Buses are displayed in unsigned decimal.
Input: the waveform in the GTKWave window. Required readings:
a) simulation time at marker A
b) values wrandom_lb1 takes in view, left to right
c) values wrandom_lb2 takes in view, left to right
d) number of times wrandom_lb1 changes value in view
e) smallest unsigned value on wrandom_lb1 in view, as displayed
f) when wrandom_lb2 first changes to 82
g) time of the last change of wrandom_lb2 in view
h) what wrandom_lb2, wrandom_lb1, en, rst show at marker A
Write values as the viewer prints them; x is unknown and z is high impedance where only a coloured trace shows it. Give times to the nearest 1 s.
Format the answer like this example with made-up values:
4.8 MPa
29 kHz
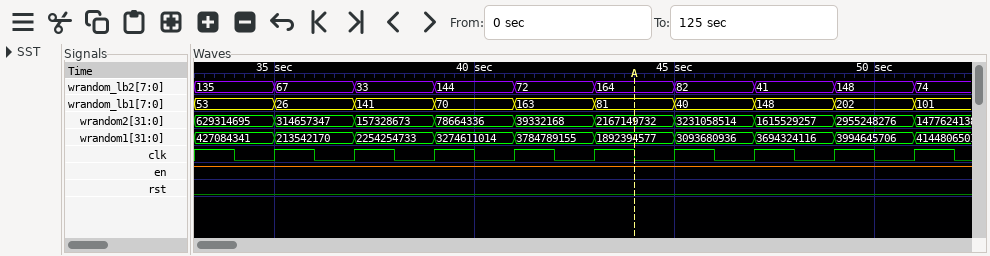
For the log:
44 s
53, 26, 141, 70, 163, 81, 40, 148, 202, 101
135, 67, 33, 144, 72, 164, 82, 41, 148, 74
9
26
45 s
51 s
wrandom_lb2=164, wrandom_lb1=81, en=1, rst=0
